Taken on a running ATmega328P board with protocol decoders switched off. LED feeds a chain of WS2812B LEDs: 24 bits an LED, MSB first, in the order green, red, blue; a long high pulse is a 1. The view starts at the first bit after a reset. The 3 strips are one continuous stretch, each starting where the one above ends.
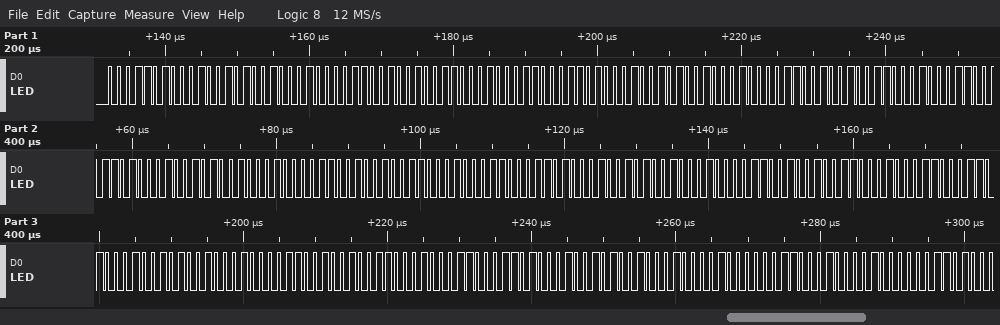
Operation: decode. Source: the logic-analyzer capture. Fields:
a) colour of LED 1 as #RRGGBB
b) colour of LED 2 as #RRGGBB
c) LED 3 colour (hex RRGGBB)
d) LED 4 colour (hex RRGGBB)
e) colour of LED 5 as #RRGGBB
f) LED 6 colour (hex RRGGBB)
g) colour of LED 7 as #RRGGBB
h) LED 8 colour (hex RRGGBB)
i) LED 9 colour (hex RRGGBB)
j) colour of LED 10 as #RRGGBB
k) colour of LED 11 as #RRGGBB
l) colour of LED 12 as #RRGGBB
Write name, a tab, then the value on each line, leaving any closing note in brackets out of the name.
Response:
colour of LED 1 as #RRGGBB	#251A22
colour of LED 2 as #RRGGBB	#261923
LED 3 colour	#251A22
LED 4 colour	#261923
colour of LED 5 as #RRGGBB	#251A22
LED 6 colour	#261923
colour of LED 7 as #RRGGBB	#251A22
LED 8 colour	#261923
LED 9 colour	#251A22
colour of LED 10 as #RRGGBB	#261923
colour of LED 11 as #RRGGBB	#251A22
colour of LED 12 as #RRGGBB	#311008
